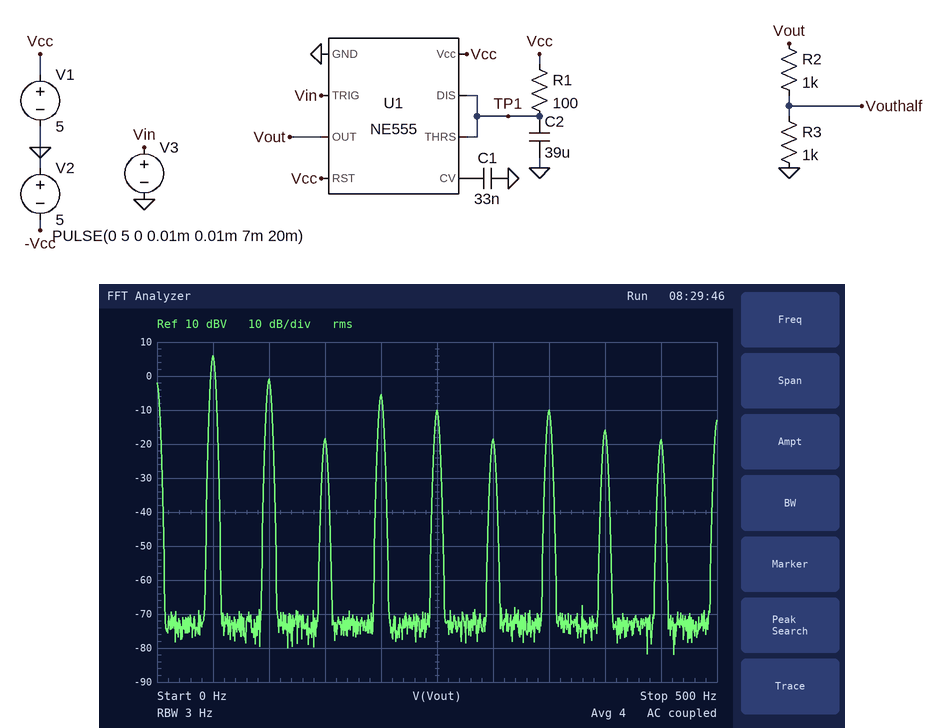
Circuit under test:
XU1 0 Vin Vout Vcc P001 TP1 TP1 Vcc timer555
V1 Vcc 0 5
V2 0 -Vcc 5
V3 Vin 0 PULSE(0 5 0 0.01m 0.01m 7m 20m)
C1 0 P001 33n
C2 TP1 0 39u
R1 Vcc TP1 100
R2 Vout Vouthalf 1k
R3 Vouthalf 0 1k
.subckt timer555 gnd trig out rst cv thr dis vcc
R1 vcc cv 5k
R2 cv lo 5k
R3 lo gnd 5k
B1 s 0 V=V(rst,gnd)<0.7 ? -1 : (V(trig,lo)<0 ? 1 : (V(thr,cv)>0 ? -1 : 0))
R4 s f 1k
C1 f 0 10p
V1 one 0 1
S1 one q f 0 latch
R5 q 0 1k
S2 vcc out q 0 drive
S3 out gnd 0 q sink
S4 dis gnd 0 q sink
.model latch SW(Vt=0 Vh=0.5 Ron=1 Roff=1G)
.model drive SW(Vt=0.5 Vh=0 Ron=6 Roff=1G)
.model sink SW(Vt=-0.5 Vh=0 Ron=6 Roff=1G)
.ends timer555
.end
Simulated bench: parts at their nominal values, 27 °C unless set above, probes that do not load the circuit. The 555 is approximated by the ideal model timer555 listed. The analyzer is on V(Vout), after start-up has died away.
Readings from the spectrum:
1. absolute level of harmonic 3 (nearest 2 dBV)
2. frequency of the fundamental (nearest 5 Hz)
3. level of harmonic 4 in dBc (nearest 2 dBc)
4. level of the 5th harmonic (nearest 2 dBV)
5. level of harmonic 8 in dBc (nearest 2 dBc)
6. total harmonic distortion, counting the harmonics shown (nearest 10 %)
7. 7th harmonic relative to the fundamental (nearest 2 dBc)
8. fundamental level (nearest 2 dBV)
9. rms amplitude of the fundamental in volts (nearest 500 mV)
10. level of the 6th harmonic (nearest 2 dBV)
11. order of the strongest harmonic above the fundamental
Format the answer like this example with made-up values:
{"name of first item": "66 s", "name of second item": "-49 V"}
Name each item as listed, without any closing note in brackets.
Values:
{"absolute level of harmonic 3": "-18 dBV", "frequency of the fundamental": "50 Hz", "level of harmonic 4 in dBc": "-12 dBc", "level of the 5th harmonic": "-10 dBV", "level of harmonic 8 in dBc": "-22 dBc", "total harmonic distortion, counting the harmonics shown": "60 %", "7th harmonic relative to the fundamental": "-16 dBc", "fundamental level": "6 dBV", "rms amplitude of the fundamental in volts": "2.0 V", "level of the 6th harmonic": "-18 dBV", "order of the strongest harmonic above the fundamental": "2"}
